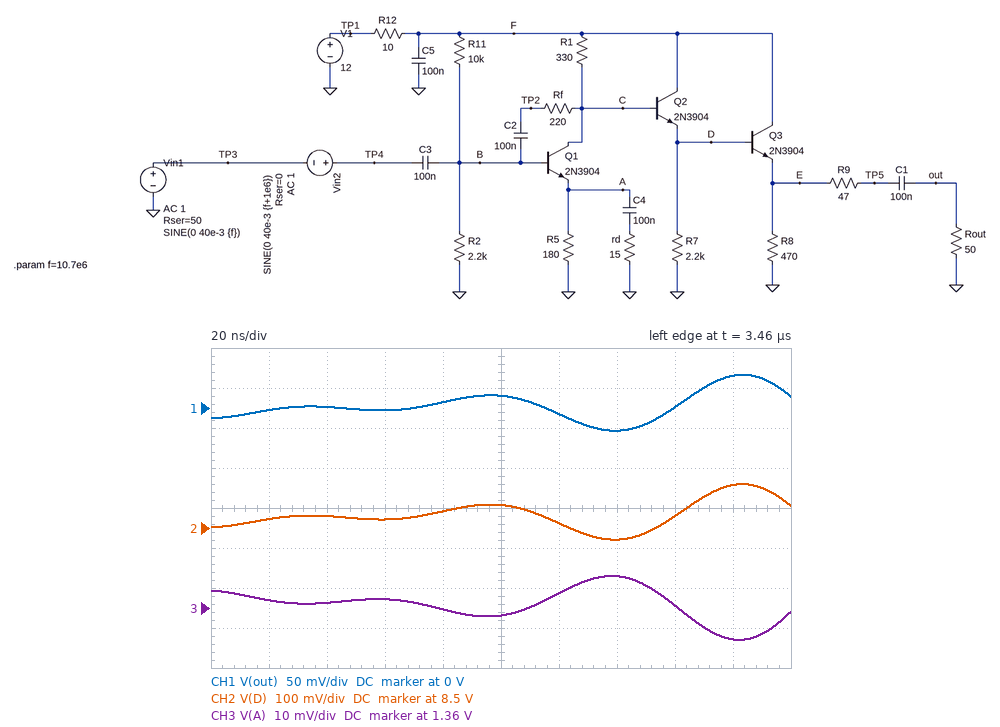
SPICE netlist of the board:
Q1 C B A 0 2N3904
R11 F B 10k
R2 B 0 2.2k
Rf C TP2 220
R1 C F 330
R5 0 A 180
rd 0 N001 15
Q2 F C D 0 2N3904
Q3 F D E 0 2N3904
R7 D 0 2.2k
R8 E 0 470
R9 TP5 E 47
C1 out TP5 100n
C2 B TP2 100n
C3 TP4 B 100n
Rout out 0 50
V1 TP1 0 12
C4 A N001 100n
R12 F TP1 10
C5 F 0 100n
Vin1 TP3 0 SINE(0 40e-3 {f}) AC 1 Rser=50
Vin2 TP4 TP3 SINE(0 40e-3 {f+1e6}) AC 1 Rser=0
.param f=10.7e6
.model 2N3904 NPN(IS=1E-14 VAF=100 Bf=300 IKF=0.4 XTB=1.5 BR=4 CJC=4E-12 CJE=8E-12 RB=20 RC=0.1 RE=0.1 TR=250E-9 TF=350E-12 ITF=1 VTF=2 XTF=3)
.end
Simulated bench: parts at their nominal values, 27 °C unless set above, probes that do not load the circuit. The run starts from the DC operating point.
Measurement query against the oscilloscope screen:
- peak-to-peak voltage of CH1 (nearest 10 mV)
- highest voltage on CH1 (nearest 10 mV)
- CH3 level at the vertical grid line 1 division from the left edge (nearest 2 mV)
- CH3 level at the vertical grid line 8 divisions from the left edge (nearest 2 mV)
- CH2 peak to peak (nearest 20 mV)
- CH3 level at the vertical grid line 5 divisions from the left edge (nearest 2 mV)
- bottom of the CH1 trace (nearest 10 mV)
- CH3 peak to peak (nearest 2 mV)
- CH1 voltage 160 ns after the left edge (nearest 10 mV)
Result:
70 mV
40 mV
1.362 V
1.360 V
140 mV
1.358 V
-30 mV
16 mV
0 V
